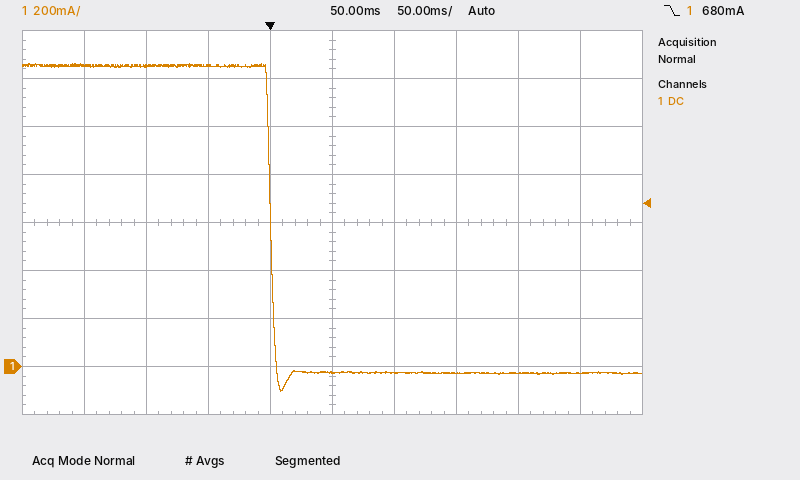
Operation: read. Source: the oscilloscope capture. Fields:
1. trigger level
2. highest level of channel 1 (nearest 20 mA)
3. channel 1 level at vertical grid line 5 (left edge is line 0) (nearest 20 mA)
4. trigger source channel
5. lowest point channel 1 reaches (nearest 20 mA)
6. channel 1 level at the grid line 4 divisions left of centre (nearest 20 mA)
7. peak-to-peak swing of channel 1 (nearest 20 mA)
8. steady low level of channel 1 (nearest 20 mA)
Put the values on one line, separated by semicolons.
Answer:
680 mA; 1.26 A; -20 mA; channel 1; -100 mA; 1.26 A; 1.36 A; -20 mA
